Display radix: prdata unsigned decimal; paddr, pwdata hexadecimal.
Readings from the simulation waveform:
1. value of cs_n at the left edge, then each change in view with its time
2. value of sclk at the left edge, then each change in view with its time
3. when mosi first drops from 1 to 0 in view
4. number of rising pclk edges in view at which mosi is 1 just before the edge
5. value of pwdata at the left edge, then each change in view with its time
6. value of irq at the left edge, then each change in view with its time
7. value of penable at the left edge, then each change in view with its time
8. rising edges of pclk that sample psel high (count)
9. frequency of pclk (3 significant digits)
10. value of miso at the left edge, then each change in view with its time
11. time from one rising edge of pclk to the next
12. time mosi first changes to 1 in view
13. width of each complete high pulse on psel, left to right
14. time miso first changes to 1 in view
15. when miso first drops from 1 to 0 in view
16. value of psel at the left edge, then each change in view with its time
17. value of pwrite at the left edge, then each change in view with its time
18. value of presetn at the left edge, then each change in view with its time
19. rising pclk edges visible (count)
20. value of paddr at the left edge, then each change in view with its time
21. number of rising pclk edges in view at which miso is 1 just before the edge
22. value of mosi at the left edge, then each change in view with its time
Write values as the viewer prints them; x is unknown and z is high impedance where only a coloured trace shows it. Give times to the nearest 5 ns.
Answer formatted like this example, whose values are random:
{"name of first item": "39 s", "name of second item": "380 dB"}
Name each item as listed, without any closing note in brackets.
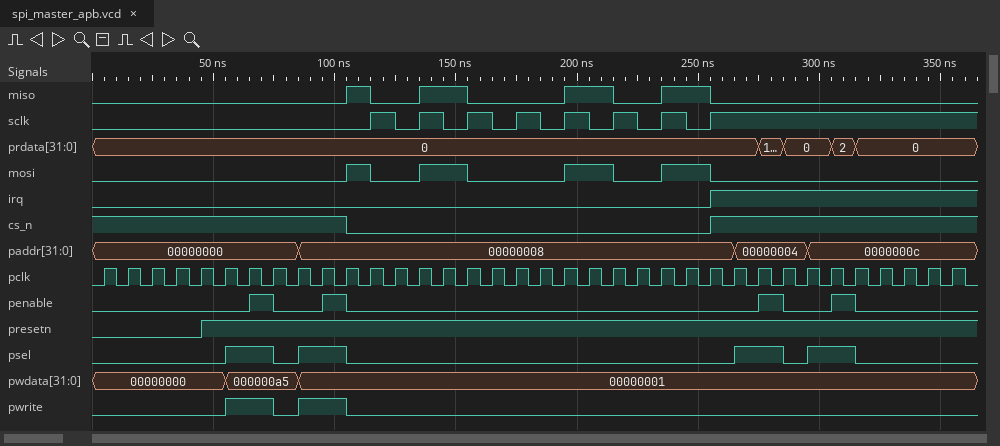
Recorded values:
{"value of cs_n at the left edge, then each change in view with its time": "1, 0 at 105 ns, 1 at 255 ns", "value of sclk at the left edge, then each change in view with its time": "0, 1 at 115 ns, 0 at 125 ns, 1 at 135 ns, 0 at 145 ns, 1 at 155 ns, 0 at 165 ns, 1 at 175 ns, 0 at 185 ns, 1 at 195 ns, 0 at 205 ns, 1 at 215 ns, 0 at 225 ns, 1 at 235 ns, 0 at 245 ns, 1 at 255 ns", "when mosi first drops from 1 to 0 in view": "115 ns", "number of rising pclk edges in view at which mosi is 1 just before the edge": "7", "value of pwdata at the left edge, then each change in view with its time": "00000000, 000000a5 at 55 ns, 00000001 at 85 ns", "value of irq at the left edge, then each change in view with its time": "0, 1 at 255 ns", "value of penable at the left edge, then each change in view with its time": "0, 1 at 65 ns, 0 at 75 ns, 1 at 95 ns, 0 at 105 ns, 1 at 275 ns, 0 at 285 ns, 1 at 305 ns, 0 at 315 ns", "rising edges of pclk that sample psel high": "8", "frequency of pclk": "100 MHz", "value of miso at the left edge, then each change in view with its time": "0, 1 at 105 ns, 0 at 115 ns, 1 at 135 ns, 0 at 155 ns, 1 at 195 ns, 0 at 215 ns, 1 at 235 ns, 0 at 255 ns", "time from one rising edge of pclk to the next": "10 ns", "time mosi first changes to 1 in view": "105 ns", "width of each complete high pulse on psel, left to right": "20 ns, 20 ns, 20 ns, 20 ns", "time miso first changes to 1 in view": "105 ns", "when miso first drops from 1 to 0 in view": "115 ns", "value of psel at the left edge, then each change in view with its time": "0, 1 at 55 ns, 0 at 75 ns, 1 at 85 ns, 0 at 105 ns, 1 at 265 ns, 0 at 285 ns, 1 at 295 ns, 0 at 315 ns", "value of pwrite at the left edge, then each change in view with its time": "0, 1 at 55 ns, 0 at 75 ns, 1 at 85 ns, 0 at 105 ns", "value of presetn at the left edge, then each change in view with its time": "0, 1 at 45 ns", "rising pclk edges visible": "36", "value of paddr at the left edge, then each change in view with its time": "00000000, 00000008 at 85 ns, 00000004 at 265 ns, 0000000c at 295 ns", "number of rising pclk edges in view at which miso is 1 just before the edge": "7", "value of mosi at the left edge, then each change in view with its time": "0, 1 at 105 ns, 0 at 115 ns, 1 at 135 ns, 0 at 155 ns, 1 at 195 ns, 0 at 215 ns, 1 at 235 ns, 0 at 255 ns"}
